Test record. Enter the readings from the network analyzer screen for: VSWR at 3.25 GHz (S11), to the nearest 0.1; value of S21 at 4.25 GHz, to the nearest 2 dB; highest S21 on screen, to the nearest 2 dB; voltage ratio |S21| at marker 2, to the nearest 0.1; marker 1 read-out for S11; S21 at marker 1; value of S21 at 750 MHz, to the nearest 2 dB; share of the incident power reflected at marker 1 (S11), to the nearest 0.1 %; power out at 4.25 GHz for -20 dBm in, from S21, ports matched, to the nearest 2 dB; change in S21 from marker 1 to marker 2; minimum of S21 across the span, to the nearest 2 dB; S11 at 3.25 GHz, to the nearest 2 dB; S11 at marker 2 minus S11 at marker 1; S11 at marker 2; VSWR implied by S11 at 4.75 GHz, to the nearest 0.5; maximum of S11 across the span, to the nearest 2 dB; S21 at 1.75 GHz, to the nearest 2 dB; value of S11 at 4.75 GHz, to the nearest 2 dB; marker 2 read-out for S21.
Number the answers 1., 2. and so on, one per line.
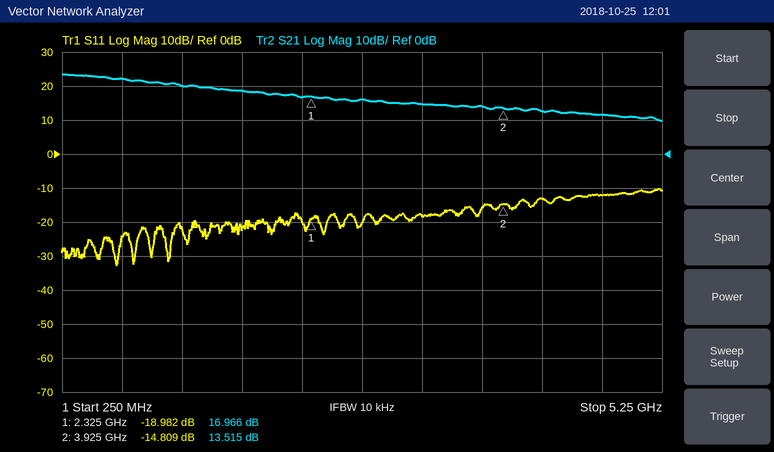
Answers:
1. 1.3
2. 12 dB
3. 24 dB
4. 4.7
5. -18.982 dB
6. 16.966 dB
7. 22 dB
8. 1.3 %
9. -8 dBm
10. -3.451 dB
11. 10 dB
12. -18 dB
13. 4.173 dB
14. -14.809 dB
15. 1.5
16. -10 dB
17. 18 dB
18. -12 dB
19. 13.515 dB
